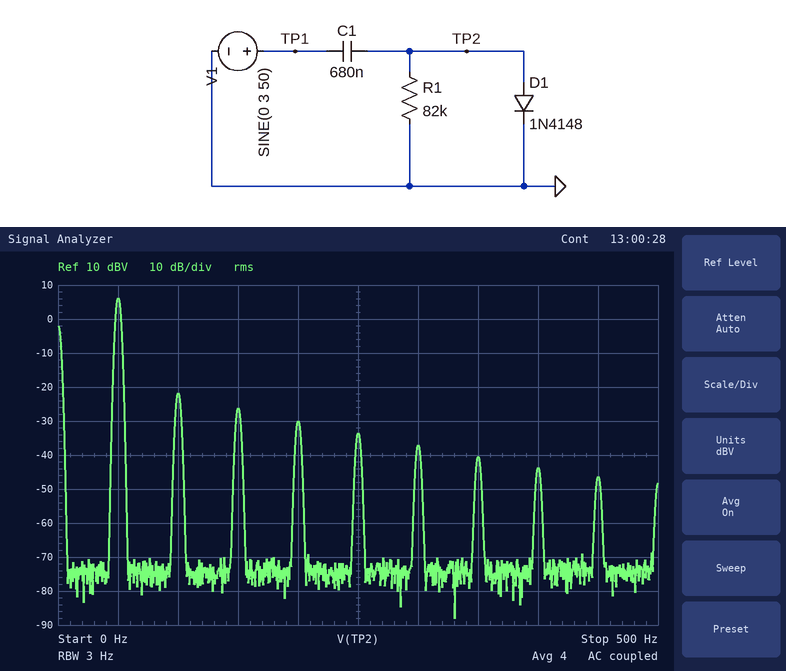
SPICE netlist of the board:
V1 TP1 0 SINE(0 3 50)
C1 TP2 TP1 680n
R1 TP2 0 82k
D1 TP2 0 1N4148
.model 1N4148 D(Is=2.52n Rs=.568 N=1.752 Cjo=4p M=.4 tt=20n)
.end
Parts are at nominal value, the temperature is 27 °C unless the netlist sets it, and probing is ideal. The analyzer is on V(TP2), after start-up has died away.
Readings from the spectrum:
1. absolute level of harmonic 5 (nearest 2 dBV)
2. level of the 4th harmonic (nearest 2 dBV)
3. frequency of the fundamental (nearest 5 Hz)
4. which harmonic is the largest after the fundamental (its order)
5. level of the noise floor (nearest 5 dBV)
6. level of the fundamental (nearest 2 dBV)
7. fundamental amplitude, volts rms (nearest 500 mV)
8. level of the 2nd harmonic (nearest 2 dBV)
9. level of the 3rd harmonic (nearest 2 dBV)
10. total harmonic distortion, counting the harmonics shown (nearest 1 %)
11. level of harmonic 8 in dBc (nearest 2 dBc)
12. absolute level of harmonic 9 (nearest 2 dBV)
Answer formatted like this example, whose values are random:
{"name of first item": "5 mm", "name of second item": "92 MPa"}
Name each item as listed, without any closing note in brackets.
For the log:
{"absolute level of harmonic 5": "-34 dBV", "level of the 4th harmonic": "-30 dBV", "frequency of the fundamental": "50 Hz", "which harmonic is the largest after the fundamental": "2", "level of the noise floor": "-75 dBV", "level of the fundamental": "6 dBV", "fundamental amplitude, volts rms": "2.0 V", "level of the 2nd harmonic": "-22 dBV", "level of the 3rd harmonic": "-26 dBV", "total harmonic distortion, counting the harmonics shown": "5 %", "level of harmonic 8 in dBc": "-50 dBc", "absolute level of harmonic 9": "-46 dBV"}
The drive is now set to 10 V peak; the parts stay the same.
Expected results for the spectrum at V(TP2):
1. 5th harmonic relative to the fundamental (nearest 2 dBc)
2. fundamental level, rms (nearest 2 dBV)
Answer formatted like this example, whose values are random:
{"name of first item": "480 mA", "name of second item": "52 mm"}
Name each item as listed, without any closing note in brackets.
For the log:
{"5th harmonic relative to the fundamental": "-38 dBc", "fundamental level, rms": "16 dBV"}
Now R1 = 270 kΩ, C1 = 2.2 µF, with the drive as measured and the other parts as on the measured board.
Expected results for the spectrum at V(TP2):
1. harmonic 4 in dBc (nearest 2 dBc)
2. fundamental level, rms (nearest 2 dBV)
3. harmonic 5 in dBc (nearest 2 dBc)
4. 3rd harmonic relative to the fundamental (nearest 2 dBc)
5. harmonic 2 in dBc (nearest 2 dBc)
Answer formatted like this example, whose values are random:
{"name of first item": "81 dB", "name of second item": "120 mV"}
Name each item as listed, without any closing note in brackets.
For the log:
{"harmonic 4 in dBc": "-54 dBc", "fundamental level, rms": "6 dBV", "harmonic 5 in dBc": "-56 dBc", "3rd harmonic relative to the fundamental": "-52 dBc", "harmonic 2 in dBc": "-48 dBc"}
